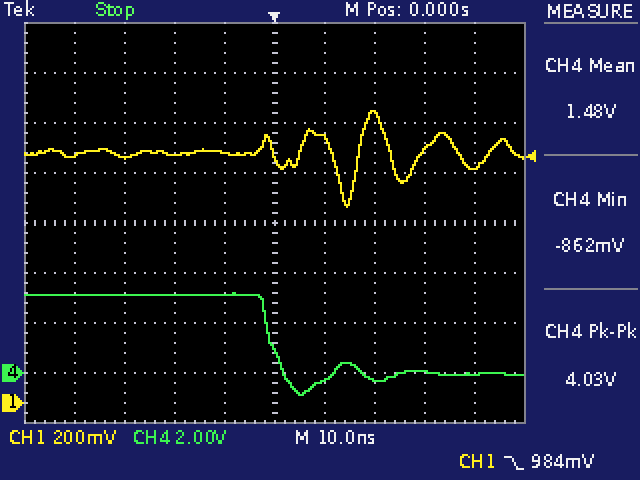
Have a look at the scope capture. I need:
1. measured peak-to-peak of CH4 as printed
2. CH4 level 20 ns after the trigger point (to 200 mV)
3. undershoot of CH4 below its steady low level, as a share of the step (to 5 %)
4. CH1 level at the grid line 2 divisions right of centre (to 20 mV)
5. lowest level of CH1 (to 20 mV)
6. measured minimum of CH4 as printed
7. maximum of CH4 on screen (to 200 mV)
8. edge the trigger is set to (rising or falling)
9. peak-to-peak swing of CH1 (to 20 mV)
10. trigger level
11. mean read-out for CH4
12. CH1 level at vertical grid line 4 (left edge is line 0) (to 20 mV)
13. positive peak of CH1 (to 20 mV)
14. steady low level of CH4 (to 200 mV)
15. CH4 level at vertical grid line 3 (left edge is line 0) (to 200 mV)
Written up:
4.03 V
-200 mV
25 %
1.16 V
780 mV
-862 mV
3.2 V
falling
380 mV
984 mV
1.48 V
1.00 V
1.16 V
0.0 V
3.2 V
